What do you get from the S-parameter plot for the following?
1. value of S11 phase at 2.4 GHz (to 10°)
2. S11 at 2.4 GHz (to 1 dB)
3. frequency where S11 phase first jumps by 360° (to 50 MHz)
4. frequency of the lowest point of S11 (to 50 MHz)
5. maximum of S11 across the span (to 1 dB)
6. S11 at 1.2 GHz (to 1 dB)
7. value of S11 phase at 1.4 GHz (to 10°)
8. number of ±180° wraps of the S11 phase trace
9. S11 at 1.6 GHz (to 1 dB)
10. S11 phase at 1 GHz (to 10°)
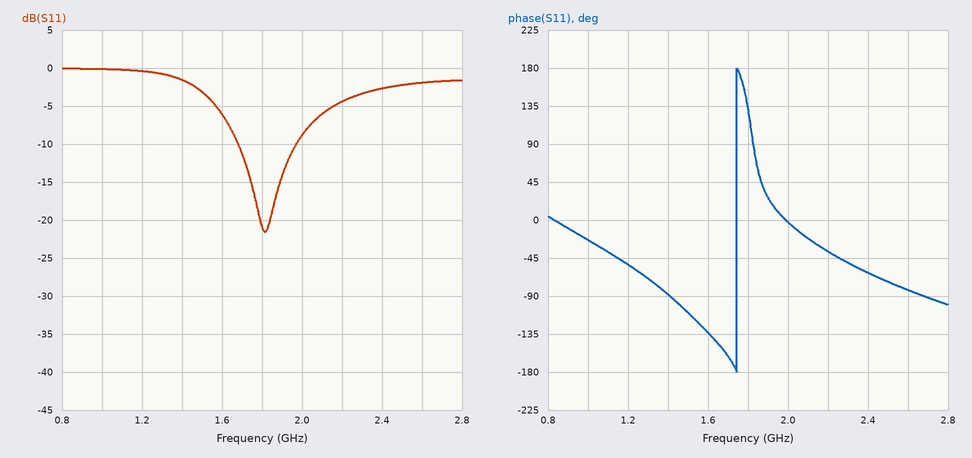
-60°
-3 dB
1.75 GHz
1.80 GHz
0 dB
0 dB
-90°
1
-6 dB
-20°
